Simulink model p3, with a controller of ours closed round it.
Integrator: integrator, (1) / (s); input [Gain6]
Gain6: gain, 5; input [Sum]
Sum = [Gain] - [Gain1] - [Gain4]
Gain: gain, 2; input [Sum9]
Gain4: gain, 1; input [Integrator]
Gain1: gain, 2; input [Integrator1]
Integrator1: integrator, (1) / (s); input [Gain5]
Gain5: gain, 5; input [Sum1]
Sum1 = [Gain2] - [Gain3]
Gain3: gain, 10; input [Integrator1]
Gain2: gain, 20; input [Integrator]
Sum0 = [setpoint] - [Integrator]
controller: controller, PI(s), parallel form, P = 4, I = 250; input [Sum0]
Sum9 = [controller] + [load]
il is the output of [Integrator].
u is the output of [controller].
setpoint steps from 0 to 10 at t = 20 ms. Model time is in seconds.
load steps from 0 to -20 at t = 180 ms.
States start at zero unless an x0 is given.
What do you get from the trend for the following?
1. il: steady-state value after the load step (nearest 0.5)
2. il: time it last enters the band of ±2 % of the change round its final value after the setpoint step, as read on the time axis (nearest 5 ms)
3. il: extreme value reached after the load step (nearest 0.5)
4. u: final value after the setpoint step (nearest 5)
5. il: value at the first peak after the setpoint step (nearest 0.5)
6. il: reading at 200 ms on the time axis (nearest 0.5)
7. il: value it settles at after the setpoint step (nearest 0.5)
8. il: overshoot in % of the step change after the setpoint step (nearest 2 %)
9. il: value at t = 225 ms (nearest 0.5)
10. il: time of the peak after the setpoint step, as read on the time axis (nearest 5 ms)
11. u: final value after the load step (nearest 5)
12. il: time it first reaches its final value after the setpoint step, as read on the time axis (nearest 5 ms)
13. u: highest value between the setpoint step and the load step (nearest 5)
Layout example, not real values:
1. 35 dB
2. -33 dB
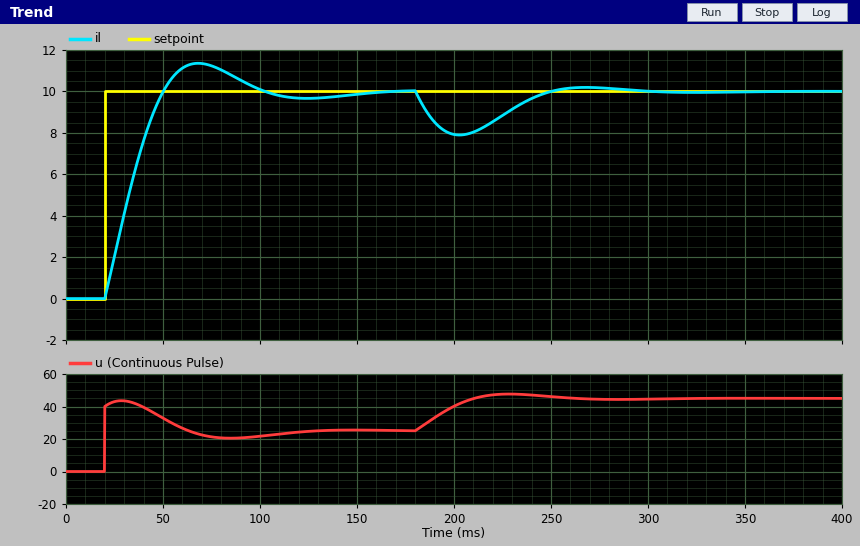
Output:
1. 10.0
2. 145 ms
3. 8.0
4. 25
5. 11.5
6. 8.0
7. 10.0
8. 14 %
9. 9.0
10. 70 ms
11. 45
12. 50 ms
13. 45
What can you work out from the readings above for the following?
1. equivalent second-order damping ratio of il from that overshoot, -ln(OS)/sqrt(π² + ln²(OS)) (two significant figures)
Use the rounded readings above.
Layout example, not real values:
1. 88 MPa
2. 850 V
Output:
1. 0.53
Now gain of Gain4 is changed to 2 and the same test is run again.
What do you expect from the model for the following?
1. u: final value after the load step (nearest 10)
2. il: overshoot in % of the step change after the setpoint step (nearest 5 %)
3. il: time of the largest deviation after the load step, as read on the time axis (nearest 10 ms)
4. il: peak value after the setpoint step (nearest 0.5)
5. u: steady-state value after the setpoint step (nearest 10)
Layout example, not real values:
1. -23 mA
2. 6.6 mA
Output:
1. 50
2. 10 %
3. 200 ms
4. 11.0
5. 30
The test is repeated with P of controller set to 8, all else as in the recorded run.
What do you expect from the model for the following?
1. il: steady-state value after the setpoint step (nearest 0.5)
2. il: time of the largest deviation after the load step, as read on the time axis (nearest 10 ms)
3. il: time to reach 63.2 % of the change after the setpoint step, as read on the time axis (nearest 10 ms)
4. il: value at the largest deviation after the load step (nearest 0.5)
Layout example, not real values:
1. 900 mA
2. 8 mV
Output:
1. 10.0
2. 200 ms
3. 30 ms
4. 8.5
